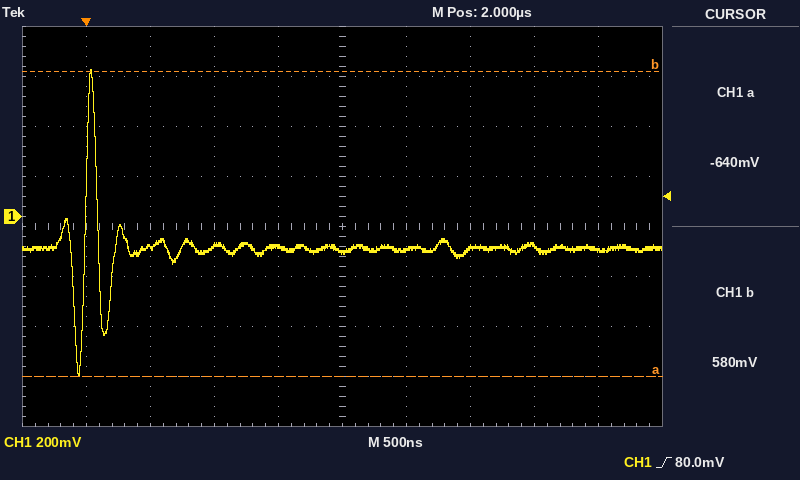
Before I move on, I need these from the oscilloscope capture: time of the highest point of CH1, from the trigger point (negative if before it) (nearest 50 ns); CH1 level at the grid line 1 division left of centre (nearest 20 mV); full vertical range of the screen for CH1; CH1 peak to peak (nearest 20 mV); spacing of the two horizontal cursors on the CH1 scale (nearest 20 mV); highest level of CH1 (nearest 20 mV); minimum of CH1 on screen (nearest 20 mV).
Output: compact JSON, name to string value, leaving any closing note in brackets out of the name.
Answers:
{"time of the highest point of CH1, from the trigger point (negative if before it)": "+50 ns", "CH1 level at the grid line 1 division left of centre": "-120 mV", "full vertical range of the screen for CH1": "1.6 V", "CH1 peak to peak": "1.22 V", "spacing of the two horizontal cursors on the CH1 scale": "1.22 V", "highest level of CH1": "580 mV", "minimum of CH1 on screen": "-640 mV"}
